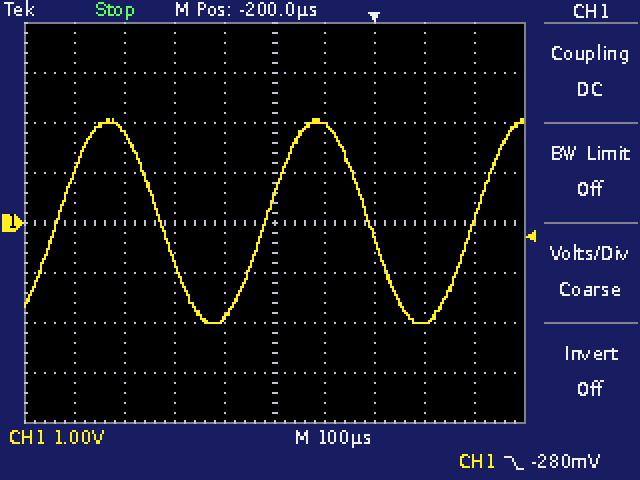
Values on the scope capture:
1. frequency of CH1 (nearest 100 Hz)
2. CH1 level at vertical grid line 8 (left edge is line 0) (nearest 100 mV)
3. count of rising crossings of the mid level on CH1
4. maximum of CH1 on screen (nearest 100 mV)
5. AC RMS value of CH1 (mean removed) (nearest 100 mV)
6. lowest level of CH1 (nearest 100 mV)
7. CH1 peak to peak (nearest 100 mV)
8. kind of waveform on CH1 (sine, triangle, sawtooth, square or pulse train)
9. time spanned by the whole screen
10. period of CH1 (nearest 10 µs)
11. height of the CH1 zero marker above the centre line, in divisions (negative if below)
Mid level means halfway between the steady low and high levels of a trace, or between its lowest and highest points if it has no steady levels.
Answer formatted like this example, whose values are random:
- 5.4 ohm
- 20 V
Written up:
- 2.4 kHz
- -2.0 V
- 3
- 2.1 V
- 1.4 V
- -2.0 V
- 4.1 V
- sine
- 1 ms
- 420 µs
- 0.0 div
